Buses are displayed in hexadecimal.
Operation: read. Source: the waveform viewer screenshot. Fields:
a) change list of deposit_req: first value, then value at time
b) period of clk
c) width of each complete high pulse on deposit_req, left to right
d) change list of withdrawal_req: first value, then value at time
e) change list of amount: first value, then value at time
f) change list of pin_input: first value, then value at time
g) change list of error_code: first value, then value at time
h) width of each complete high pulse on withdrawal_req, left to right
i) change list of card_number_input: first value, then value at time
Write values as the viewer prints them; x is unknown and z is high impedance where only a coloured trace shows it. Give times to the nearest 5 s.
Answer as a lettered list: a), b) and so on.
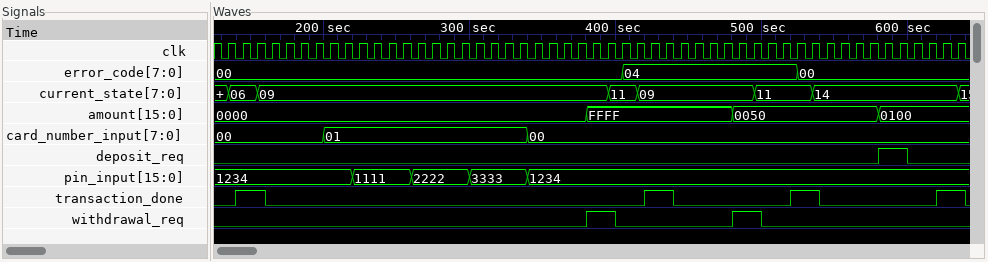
a) 0, 1 at 580 s, 0 at 600 s
b) 10 s
c) 20 s
d) 0, 1 at 380 s, 0 at 400 s, 1 at 480 s, 0 at 500 s
e) 0000, FFFF at 380 s, 0050 at 480 s, 0100 at 580 s
f) 1234, 1111 at 220 s, 2222 at 260 s, 3333 at 300 s, 1234 at 340 s
g) 00, 04 at 405 s, 00 at 525 s
h) 20 s, 20 s
i) 00, 01 at 200 s, 00 at 340 s
